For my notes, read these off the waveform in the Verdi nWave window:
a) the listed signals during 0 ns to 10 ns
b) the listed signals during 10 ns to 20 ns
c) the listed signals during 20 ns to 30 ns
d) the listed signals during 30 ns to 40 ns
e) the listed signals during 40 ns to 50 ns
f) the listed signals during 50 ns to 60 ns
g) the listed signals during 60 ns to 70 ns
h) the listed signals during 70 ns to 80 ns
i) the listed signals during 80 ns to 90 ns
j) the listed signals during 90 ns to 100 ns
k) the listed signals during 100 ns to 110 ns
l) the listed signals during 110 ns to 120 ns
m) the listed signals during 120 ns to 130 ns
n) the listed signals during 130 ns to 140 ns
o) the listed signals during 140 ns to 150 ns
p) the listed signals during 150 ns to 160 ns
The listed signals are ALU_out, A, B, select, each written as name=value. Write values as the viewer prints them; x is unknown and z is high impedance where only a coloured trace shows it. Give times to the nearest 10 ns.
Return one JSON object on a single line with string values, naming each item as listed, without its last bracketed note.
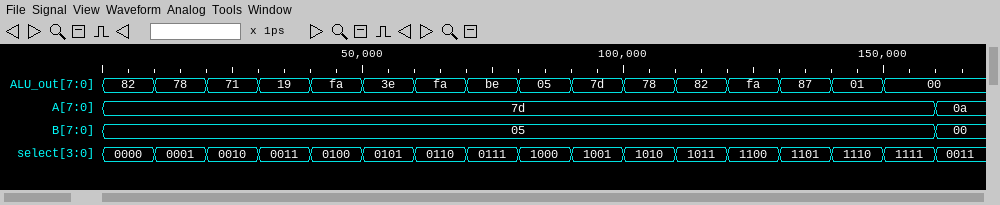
{"the listed signals during 0 ns to 10 ns": "ALU_out=82, A=7d, B=05, select=0000", "the listed signals during 10 ns to 20 ns": "ALU_out=78, A=7d, B=05, select=0001", "the listed signals during 20 ns to 30 ns": "ALU_out=71, A=7d, B=05, select=0010", "the listed signals during 30 ns to 40 ns": "ALU_out=19, A=7d, B=05, select=0011", "the listed signals during 40 ns to 50 ns": "ALU_out=fa, A=7d, B=05, select=0100", "the listed signals during 50 ns to 60 ns": "ALU_out=3e, A=7d, B=05, select=0101", "the listed signals during 60 ns to 70 ns": "ALU_out=fa, A=7d, B=05, select=0110", "the listed signals during 70 ns to 80 ns": "ALU_out=be, A=7d, B=05, select=0111", "the listed signals during 80 ns to 90 ns": "ALU_out=05, A=7d, B=05, select=1000", "the listed signals during 90 ns to 100 ns": "ALU_out=7d, A=7d, B=05, select=1001", "the listed signals during 100 ns to 110 ns": "ALU_out=78, A=7d, B=05, select=1010", "the listed signals during 110 ns to 120 ns": "ALU_out=82, A=7d, B=05, select=1011", "the listed signals during 120 ns to 130 ns": "ALU_out=fa, A=7d, B=05, select=1100", "the listed signals during 130 ns to 140 ns": "ALU_out=87, A=7d, B=05, select=1101", "the listed signals during 140 ns to 150 ns": "ALU_out=01, A=7d, B=05, select=1110", "the listed signals during 150 ns to 160 ns": "ALU_out=00, A=7d, B=05, select=1111"}
